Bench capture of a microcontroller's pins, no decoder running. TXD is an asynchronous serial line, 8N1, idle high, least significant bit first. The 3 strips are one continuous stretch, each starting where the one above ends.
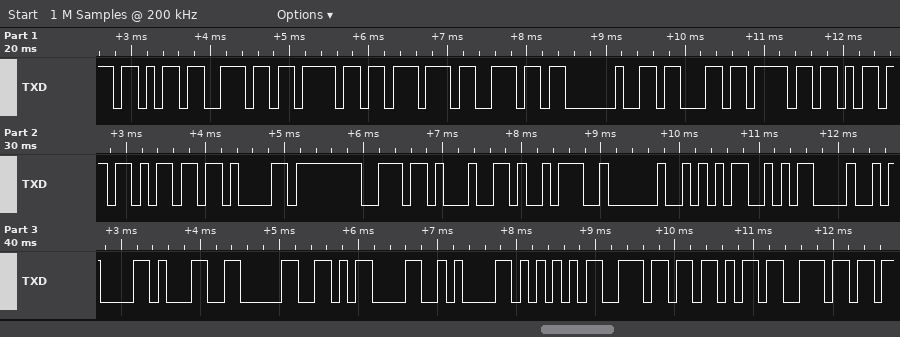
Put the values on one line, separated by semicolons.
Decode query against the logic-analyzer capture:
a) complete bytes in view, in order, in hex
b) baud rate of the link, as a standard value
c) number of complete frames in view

6B 6E 6F 77 6E 20 63 6F 6D 6D 61 6E 64 3A 20 35 0D 0A 31 30 0D 0A 55 6E 6B 6E; 9600 baud; 26
